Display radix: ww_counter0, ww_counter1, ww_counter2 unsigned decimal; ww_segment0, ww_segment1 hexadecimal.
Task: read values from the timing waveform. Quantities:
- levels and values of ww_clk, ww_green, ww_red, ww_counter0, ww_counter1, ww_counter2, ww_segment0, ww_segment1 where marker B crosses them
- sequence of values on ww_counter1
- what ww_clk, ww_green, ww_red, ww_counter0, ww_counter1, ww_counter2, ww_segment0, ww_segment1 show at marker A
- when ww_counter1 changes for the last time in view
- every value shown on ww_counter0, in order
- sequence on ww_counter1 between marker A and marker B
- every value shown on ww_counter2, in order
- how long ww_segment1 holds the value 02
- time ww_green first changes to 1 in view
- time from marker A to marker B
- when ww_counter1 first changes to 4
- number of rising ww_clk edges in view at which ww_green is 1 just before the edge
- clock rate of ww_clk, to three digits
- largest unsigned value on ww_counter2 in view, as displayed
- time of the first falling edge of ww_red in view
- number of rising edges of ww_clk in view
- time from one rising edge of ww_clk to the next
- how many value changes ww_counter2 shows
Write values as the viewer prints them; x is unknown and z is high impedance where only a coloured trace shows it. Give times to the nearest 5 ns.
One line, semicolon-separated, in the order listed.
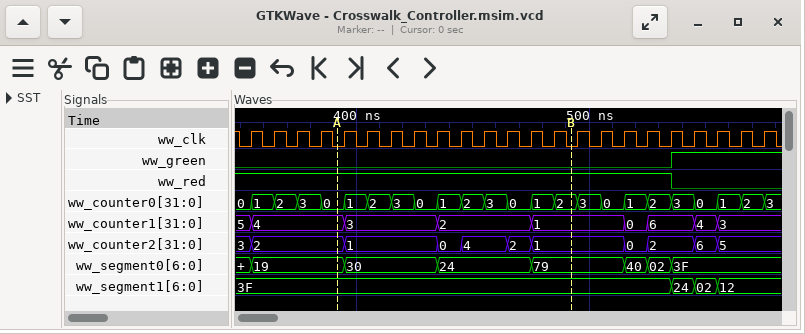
ww_clk=0, ww_green=0, ww_red=1, ww_counter0=2, ww_counter1=1, ww_counter2=1, ww_segment0=79, ww_segment1=3F; 5, 4, 3, 2, 1, 0, 6, 4, 3; ww_clk=0, ww_green=0, ww_red=1, ww_counter0=0, ww_counter1=4, ww_counter2=2, ww_segment0=19, ww_segment1=3F; 555 ns; 0, 1, 2, 3, 0, 1, 2, 3, 0, 1, 2, 3, 0, 1, 2, 3, 0, 1, 2, 3, 0, 1, 2, 3; 4, 3, 2, 1; 3, 2, 1, 0, 4, 2, 1, 0, 2, 6, 5; 10 ns; 535 ns; 100 ns; 355 ns; 4; 100 MHz; 6; 535 ns; 23; 10 ns; 10
